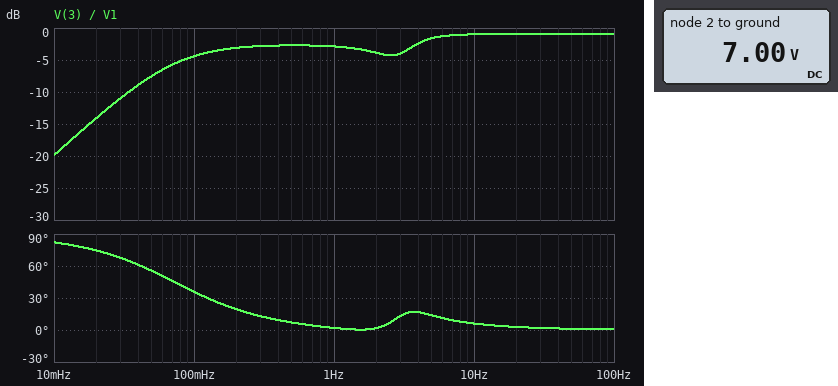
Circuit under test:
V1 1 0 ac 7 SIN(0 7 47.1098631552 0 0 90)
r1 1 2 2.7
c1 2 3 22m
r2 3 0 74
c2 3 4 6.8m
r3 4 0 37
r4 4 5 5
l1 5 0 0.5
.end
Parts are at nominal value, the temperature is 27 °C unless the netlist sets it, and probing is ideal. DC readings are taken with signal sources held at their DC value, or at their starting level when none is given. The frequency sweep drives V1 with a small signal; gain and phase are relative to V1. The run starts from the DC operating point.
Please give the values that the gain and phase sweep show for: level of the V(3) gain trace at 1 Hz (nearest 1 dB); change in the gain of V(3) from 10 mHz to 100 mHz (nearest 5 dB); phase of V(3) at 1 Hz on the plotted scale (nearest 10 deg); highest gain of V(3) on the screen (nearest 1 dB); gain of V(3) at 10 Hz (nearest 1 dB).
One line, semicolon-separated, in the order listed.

-3 dB; 15 dB; 0 deg; -1 dB; -1 dB
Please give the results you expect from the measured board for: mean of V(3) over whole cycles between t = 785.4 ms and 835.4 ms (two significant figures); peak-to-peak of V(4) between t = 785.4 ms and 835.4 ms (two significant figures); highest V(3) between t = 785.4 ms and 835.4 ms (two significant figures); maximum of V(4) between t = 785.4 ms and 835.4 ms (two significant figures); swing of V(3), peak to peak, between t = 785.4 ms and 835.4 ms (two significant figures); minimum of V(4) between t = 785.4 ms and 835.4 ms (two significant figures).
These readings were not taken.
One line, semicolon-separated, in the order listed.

-3.6 V; 13 V; 2.7 V; 6.4 V; 13 V; -6.3 V
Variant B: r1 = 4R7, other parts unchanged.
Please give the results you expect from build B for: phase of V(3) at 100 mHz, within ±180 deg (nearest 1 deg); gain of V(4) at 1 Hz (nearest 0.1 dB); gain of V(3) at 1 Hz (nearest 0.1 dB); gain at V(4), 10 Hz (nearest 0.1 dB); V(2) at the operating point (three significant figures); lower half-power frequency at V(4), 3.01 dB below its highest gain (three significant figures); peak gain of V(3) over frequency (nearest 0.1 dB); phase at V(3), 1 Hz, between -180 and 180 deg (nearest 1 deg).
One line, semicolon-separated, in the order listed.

35 deg; -15.5 dB; -3.2 dB; -1.2 dB; 7.00 V; 2.54 Hz; -1.5 dB; -2 deg
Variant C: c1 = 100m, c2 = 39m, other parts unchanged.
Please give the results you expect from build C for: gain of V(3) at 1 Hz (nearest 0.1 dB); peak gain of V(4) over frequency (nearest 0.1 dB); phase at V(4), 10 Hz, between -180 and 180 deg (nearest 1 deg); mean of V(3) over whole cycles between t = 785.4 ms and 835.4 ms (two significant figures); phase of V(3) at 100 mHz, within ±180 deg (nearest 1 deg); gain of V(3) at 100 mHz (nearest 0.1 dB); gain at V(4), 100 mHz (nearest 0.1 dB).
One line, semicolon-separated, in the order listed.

-4.5 dB; -0.9 dB; 5 deg; -4.6 V; 8 deg; -3.2 dB; -22.5 dB
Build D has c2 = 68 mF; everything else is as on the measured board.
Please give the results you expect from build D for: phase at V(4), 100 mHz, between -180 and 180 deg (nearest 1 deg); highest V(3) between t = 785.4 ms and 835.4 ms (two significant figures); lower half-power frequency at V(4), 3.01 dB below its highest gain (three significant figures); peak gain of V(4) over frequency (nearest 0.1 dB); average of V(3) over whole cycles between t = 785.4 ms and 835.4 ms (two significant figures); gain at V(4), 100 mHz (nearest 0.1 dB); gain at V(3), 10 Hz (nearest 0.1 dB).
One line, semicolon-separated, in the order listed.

102 deg; 4.9 V; 1.36 Hz; -0.6 dB; -1.4 V; -27.3 dB; -0.9 dB
